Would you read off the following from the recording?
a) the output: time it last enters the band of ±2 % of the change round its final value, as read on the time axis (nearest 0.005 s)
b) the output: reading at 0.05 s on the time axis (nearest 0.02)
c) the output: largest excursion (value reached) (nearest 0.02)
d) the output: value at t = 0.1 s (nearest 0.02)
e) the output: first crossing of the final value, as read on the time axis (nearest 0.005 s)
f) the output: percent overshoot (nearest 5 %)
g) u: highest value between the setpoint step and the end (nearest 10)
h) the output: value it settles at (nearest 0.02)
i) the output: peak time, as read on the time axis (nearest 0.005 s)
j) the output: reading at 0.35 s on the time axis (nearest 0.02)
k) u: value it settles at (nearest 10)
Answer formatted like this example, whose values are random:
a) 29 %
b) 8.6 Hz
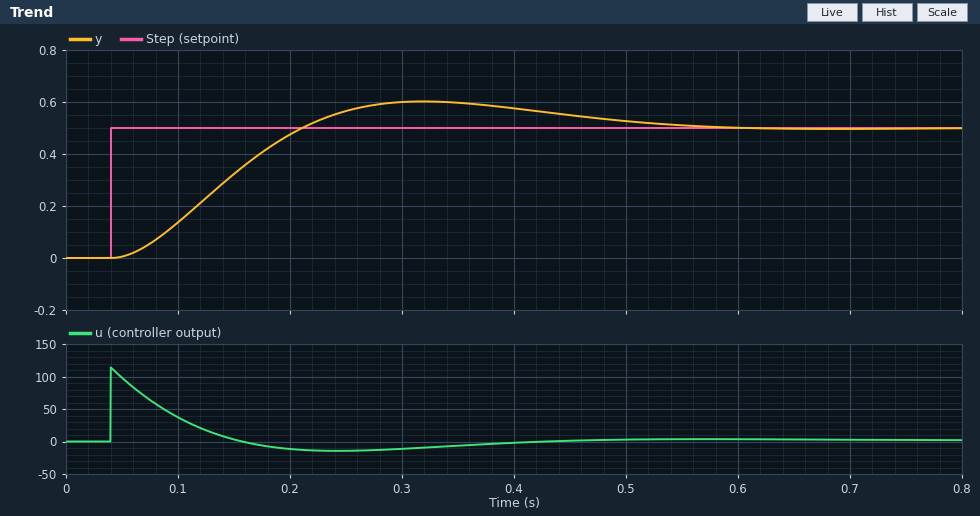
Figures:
a) 0.550 s
b) 0.00
c) 0.60
d) 0.14
e) 0.210 s
f) 20 %
g) 110
h) 0.50
i) 0.320 s
j) 0.60
k) 0
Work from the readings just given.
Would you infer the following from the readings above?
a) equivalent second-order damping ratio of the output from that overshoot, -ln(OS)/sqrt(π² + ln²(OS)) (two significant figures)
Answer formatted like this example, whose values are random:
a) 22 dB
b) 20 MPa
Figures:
a) 0.46
